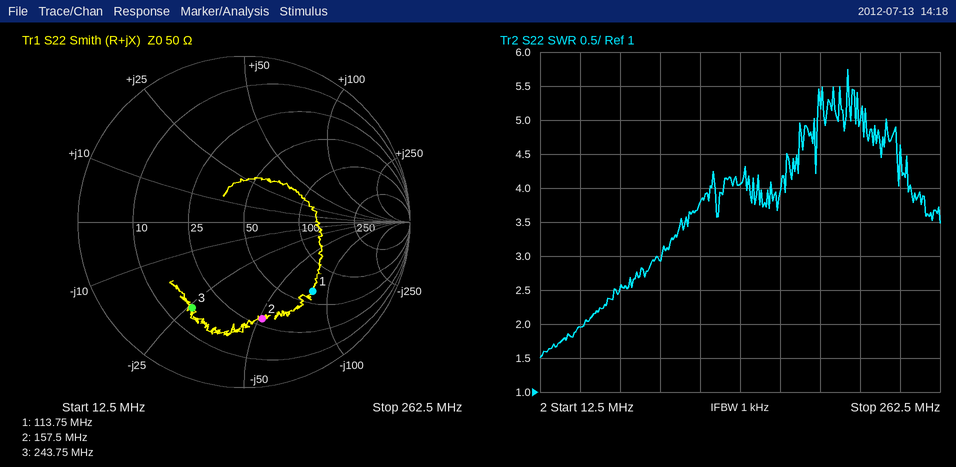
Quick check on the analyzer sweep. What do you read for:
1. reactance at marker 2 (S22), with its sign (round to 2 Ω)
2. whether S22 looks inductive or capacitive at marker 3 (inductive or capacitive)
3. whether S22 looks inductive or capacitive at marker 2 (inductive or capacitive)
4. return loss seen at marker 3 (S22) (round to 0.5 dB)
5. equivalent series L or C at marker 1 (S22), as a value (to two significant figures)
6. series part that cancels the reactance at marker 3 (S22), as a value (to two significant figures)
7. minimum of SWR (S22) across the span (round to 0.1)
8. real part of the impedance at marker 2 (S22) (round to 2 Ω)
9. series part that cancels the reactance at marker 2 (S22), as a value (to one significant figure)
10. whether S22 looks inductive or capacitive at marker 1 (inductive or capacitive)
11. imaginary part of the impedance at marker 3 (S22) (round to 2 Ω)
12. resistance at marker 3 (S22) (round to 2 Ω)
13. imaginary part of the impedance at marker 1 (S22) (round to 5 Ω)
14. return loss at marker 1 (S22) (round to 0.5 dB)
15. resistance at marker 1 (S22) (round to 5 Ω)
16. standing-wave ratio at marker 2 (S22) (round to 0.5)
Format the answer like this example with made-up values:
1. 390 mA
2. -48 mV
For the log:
1. -52 Ω
2. capacitive
3. capacitive
4. 4.5 dB
5. 17 pF
6. 17 nH
7. 1.5
8. 28 Ω
9. 50 nH
10. capacitive
11. -26 Ω
12. 16 Ω
13. -80 Ω
14. 4.5 dB
15. 65 Ω
16. 4.0
